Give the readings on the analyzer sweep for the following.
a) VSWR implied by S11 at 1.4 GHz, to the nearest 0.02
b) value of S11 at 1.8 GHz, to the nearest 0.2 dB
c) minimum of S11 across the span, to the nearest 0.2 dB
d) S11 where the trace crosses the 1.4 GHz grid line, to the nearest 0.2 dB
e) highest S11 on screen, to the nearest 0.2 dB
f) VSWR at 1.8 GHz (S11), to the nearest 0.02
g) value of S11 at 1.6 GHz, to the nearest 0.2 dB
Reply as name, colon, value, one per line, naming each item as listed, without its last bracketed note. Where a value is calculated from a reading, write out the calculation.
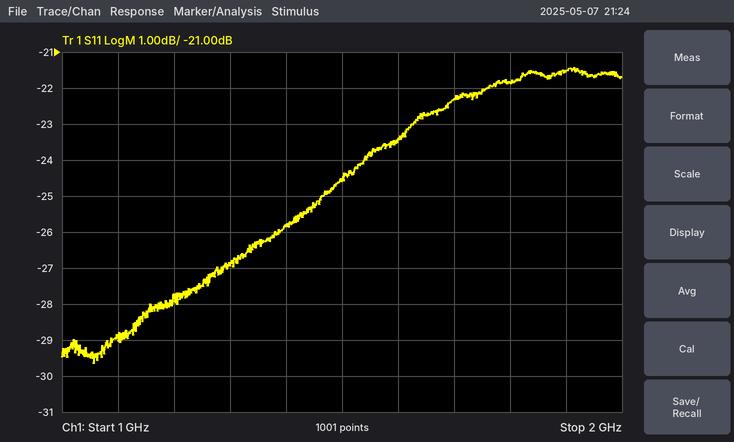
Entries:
VSWR implied by S11 at 1.4 GHz, to the nearest 0.02: |Γ| = 10^(-25.8/20) = 0.0513; VSWR = (1 + 0.0513)/(1 − 0.0513) ≈ 1.11, so 1.10 to the nearest 0.02
value of S11 at 1.8 GHz, to the nearest 0.2 dB: -21.8 dB
minimum of S11 across the span, to the nearest 0.2 dB: -29.6 dB
S11 where the trace crosses the 1.4 GHz grid line, to the nearest 0.2 dB: -25.8 dB
highest S11 on screen, to the nearest 0.2 dB: -21.4 dB
VSWR at 1.8 GHz (S11), to the nearest 0.02: |Γ| = 10^(-21.8/20) = 0.0813; VSWR = (1 + 0.0813)/(1 − 0.0813) ≈ 1.18
value of S11 at 1.6 GHz, to the nearest 0.2 dB: -23.4 dB
